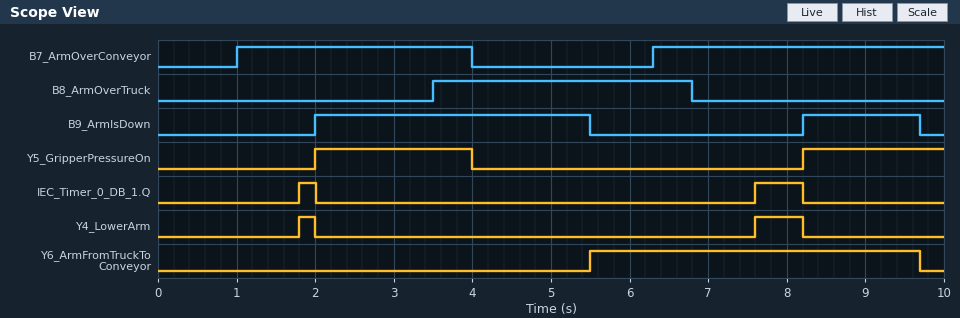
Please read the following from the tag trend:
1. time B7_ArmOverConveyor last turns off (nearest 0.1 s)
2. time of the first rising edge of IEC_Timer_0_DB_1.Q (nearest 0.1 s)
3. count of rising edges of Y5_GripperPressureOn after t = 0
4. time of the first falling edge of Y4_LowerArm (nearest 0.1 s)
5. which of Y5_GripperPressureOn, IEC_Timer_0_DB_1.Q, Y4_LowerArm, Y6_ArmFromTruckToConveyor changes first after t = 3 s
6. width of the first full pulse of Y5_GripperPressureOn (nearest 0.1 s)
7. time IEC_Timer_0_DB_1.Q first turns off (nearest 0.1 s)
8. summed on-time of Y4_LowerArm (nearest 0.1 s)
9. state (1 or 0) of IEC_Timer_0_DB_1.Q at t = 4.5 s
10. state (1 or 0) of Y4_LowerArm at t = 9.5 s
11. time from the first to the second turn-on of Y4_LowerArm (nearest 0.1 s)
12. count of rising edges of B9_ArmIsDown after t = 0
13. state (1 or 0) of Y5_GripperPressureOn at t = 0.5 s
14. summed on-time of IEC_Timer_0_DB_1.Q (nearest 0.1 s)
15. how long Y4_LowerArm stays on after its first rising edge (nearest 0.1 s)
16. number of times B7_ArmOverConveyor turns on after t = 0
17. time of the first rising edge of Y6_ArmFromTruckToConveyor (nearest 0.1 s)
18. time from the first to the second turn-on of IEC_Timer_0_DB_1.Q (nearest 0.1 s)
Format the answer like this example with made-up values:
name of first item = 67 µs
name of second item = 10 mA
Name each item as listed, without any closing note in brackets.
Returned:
time B7_ArmOverConveyor last turns off = 4.0 s
time of the first rising edge of IEC_Timer_0_DB_1.Q = 1.8 s
count of rising edges of Y5_GripperPressureOn after t = 0 = 2
time of the first falling edge of Y4_LowerArm = 2.0 s
which of Y5_GripperPressureOn, IEC_Timer_0_DB_1.Q, Y4_LowerArm, Y6_ArmFromTruckToConveyor changes first after t = 3 s = Y5_GripperPressureOn
width of the first full pulse of Y5_GripperPressureOn = 2.0 s
time IEC_Timer_0_DB_1.Q first turns off = 2.0 s
summed on-time of Y4_LowerArm = 0.8 s
state (1 or 0) of IEC_Timer_0_DB_1.Q at t = 4.5 s = 0
state (1 or 0) of Y4_LowerArm at t = 9.5 s = 0
time from the first to the second turn-on of Y4_LowerArm = 5.8 s
count of rising edges of B9_ArmIsDown after t = 0 = 2
state (1 or 0) of Y5_GripperPressureOn at t = 0.5 s = 0
summed on-time of IEC_Timer_0_DB_1.Q = 0.8 s
how long Y4_LowerArm stays on after its first rising edge = 0.2 s
number of times B7_ArmOverConveyor turns on after t = 0 = 2
time of the first rising edge of Y6_ArmFromTruckToConveyor = 5.5 s
time from the first to the second turn-on of IEC_Timer_0_DB_1.Q = 5.8 s
